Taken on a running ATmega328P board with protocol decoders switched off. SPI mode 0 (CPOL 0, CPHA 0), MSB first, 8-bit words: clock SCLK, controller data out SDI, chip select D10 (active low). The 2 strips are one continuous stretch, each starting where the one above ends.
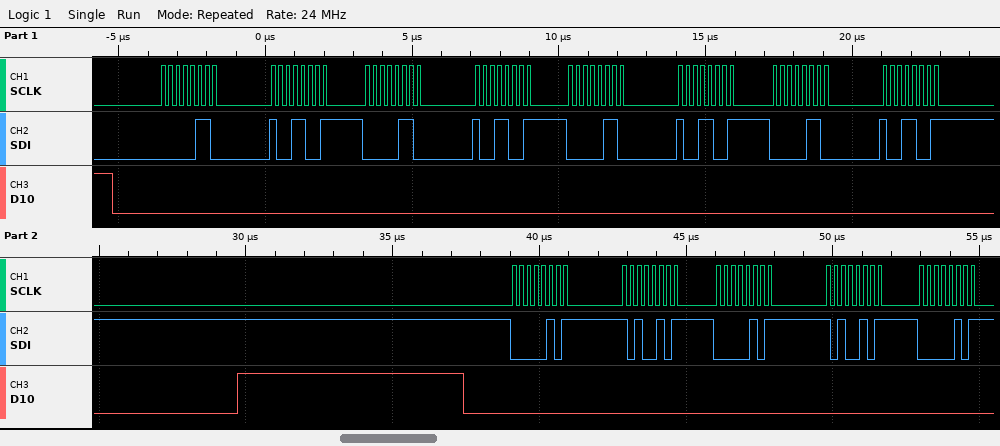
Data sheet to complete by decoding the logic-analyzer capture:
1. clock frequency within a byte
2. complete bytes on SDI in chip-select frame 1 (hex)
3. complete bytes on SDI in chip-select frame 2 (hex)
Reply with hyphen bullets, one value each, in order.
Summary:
- 4 MHz
- 06 99 06 99 06 99 06 99
- 05 A5 05 A5 05
